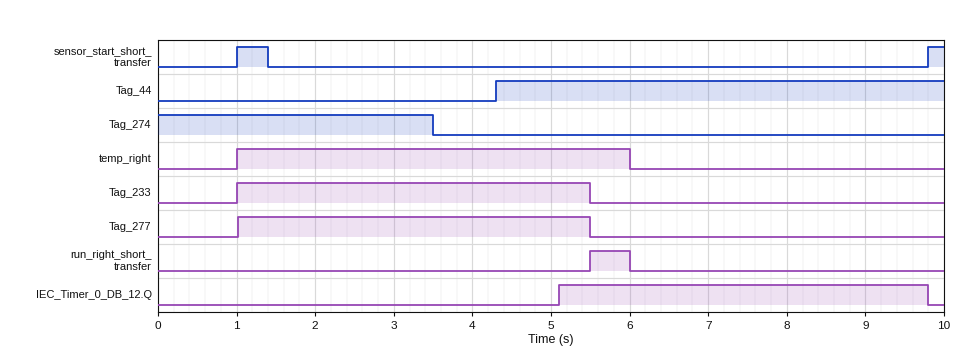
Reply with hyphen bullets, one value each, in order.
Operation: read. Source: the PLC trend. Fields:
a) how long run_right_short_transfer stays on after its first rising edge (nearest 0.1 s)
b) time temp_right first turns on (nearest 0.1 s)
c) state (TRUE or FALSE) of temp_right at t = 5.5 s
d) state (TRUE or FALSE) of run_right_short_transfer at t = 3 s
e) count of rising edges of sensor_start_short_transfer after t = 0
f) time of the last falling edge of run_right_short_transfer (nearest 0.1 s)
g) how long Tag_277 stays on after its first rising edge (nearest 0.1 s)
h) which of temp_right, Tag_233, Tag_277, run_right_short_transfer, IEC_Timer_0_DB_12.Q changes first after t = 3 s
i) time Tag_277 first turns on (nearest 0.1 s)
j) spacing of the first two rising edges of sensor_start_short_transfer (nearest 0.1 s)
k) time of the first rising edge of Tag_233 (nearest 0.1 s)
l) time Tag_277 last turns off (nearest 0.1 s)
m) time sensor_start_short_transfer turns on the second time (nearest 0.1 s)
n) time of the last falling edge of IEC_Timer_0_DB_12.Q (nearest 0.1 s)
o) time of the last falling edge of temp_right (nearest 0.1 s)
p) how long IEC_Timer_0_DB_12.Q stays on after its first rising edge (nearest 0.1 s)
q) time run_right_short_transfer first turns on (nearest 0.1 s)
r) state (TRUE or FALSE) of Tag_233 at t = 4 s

- 0.5 s
- 1.0 s
- TRUE
- FALSE
- 2
- 6.0 s
- 4.5 s
- IEC_Timer_0_DB_12.Q
- 1.0 s
- 8.8 s
- 1.0 s
- 5.5 s
- 9.8 s
- 9.8 s
- 6.0 s
- 4.7 s
- 5.5 s
- TRUE
